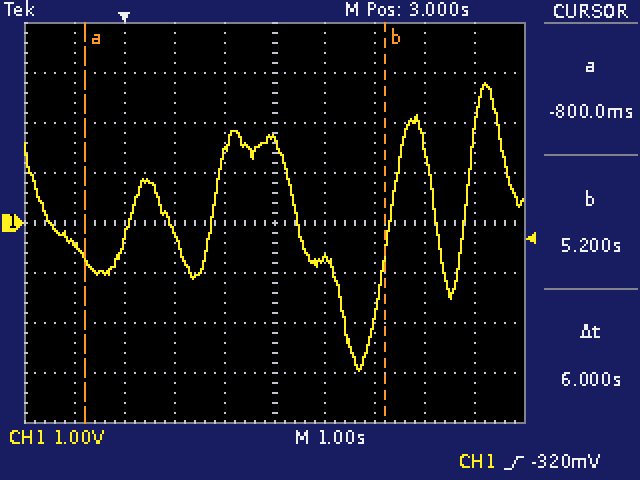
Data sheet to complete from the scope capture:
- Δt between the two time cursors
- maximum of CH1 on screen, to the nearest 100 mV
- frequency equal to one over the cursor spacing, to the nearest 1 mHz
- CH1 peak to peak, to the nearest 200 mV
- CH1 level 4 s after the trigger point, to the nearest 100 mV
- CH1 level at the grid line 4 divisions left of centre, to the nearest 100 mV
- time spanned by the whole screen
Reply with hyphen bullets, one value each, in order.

- 6 s
- 2.8 V
- 167 mHz
- 5.8 V
- -700 mV
- -400 mV
- 10 s
